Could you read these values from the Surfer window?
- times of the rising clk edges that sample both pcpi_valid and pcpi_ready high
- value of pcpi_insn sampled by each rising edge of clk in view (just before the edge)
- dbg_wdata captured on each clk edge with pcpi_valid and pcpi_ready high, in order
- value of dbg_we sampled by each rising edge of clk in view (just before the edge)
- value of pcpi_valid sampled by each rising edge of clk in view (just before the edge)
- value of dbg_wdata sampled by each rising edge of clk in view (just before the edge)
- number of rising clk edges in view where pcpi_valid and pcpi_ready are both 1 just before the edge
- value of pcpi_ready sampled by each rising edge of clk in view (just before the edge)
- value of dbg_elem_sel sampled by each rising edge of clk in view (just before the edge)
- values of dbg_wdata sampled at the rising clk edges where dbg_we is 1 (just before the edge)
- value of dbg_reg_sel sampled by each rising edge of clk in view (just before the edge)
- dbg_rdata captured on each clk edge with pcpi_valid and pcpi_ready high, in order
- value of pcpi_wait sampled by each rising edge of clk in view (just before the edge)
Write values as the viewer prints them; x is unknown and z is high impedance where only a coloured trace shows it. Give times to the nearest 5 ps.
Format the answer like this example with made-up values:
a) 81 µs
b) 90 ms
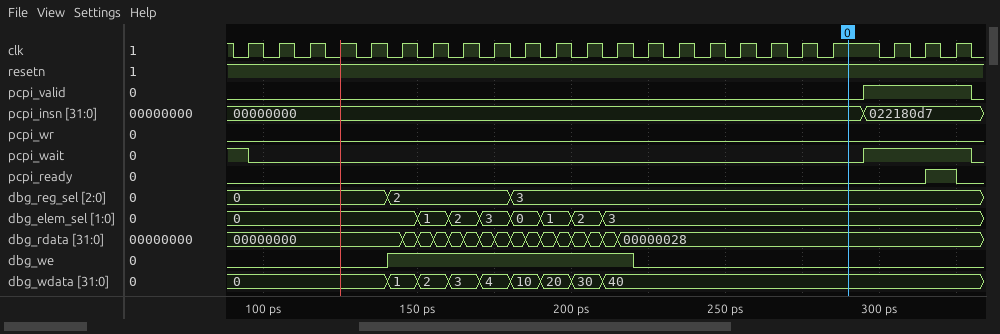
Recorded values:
a) 325 ps
b) 00000000, 00000000, 00000000, 00000000, 00000000, 00000000, 00000000, 00000000, 00000000, 00000000, 00000000, 00000000, 00000000, 00000000, 00000000, 00000000, 00000000, 00000000, 00000000, 00000000, 022180d7, 022180d7, 022180d7
c) 40
d) 0 0 0 0 0 1 1 1 1 1 1 1 1 0 0 0 0 0 0 0 0 0 0
e) 0 0 0 0 0 0 0 0 0 0 0 0 0 0 0 0 0 0 0 0 1 1 1
f) 0, 0, 0, 0, 0, 1, 2, 3, 4, 10, 20, 30, 40, 40, 40, 40, 40, 40, 40, 40, 40, 40, 40
g) 1
h) 0 0 0 0 0 0 0 0 0 0 0 0 0 0 0 0 0 0 0 0 0 0 1
i) 0, 0, 0, 0, 0, 0, 1, 2, 3, 0, 1, 2, 3, 3, 3, 3, 3, 3, 3, 3, 3, 3, 3
j) 1, 2, 3, 4, 10, 20, 30, 40
k) 0, 0, 0, 0, 0, 2, 2, 2, 2, 3, 3, 3, 3, 3, 3, 3, 3, 3, 3, 3, 3, 3, 3
l) 00000028
m) 1 0 0 0 0 0 0 0 0 0 0 0 0 0 0 0 0 0 0 0 1 1 1
